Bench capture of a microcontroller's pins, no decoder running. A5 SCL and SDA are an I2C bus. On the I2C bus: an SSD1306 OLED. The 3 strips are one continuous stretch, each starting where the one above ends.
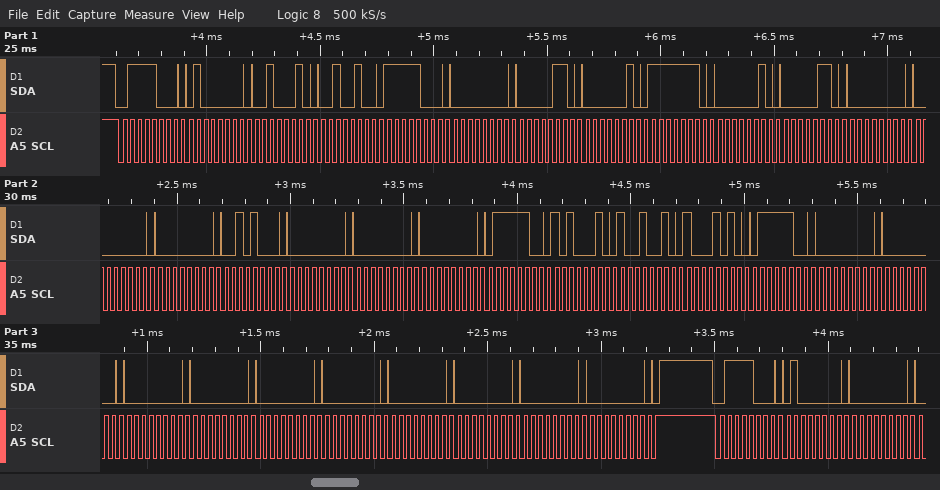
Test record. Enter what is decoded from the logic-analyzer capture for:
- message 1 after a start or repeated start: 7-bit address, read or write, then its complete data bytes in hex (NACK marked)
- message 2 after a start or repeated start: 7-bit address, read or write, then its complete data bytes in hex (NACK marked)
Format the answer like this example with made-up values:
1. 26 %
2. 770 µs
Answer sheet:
1. 0x3C write: 40 22 24 F8 00 06 02 FE 02 06 00 00 00 28 00 00 00 7C A2 92 8A 7C 00 00 00 00 00 00 00 00 00 00
2. 0x3C write: 40 00
